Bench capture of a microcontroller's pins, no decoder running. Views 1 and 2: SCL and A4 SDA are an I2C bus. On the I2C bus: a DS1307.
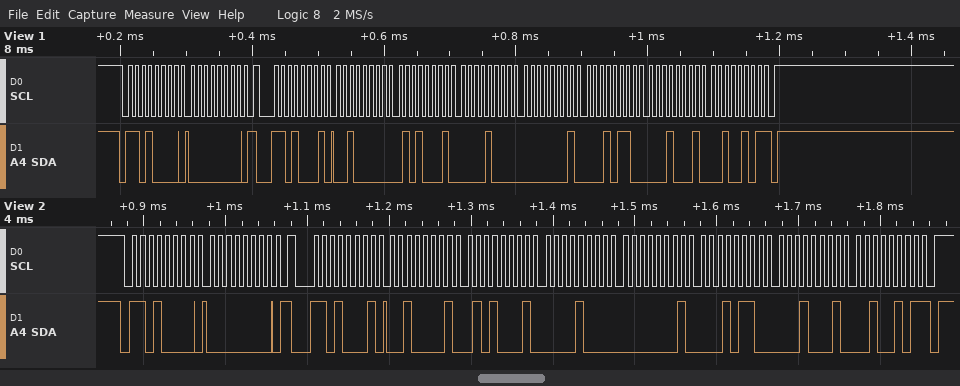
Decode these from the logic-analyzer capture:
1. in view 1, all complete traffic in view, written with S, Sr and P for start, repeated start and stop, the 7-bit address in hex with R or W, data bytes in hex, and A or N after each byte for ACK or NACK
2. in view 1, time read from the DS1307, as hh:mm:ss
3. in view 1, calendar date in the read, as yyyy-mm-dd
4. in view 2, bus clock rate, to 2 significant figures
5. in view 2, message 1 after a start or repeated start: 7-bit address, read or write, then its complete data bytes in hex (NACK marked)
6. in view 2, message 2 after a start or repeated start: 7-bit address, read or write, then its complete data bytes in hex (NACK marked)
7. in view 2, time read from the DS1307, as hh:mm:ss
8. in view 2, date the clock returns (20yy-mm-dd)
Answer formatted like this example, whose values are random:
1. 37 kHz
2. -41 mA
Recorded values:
1. S 68W A 00 A Sr 68R A 20 A 51 A 08 A 01 A 16 A 11 A 25 N P
2. 08:51:20
3. 2025-11-16
4. 100 kHz
5. 0x68 write: 00
6. 0x68 read: 21 51 08 01 16 11 25 NACK
7. 08:51:21
8. 2025-11-16
